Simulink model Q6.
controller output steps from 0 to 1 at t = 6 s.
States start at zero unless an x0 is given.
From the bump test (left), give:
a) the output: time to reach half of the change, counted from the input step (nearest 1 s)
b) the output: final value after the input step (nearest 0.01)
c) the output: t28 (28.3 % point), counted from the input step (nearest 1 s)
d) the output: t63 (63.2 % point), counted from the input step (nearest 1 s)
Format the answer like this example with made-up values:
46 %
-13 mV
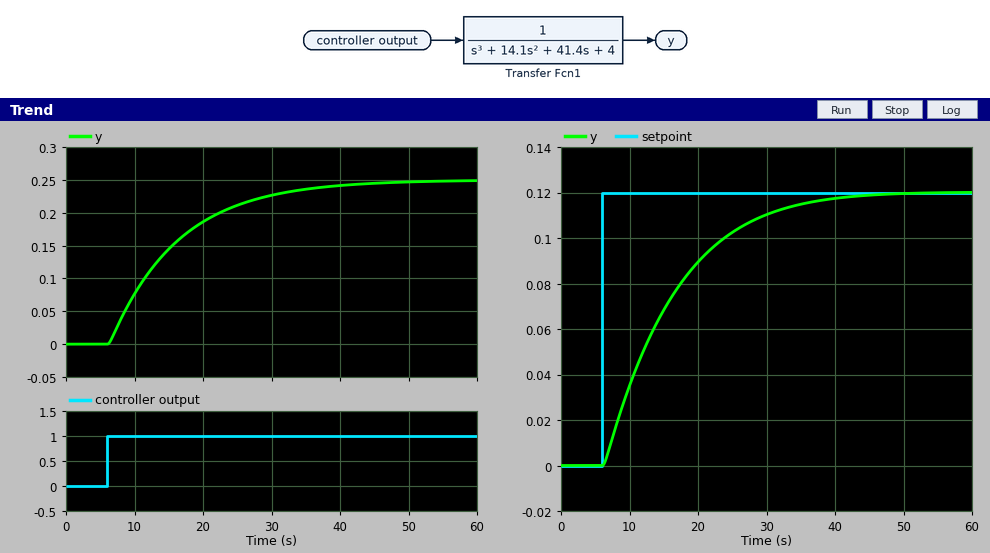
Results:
7 s
0.25
4 s
10 s
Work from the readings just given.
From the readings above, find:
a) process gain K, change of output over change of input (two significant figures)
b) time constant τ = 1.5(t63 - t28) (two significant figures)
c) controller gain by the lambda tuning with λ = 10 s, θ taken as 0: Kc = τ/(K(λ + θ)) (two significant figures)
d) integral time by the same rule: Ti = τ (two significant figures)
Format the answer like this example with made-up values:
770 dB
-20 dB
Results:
0.25
9.0 s
3.6
9.0 s
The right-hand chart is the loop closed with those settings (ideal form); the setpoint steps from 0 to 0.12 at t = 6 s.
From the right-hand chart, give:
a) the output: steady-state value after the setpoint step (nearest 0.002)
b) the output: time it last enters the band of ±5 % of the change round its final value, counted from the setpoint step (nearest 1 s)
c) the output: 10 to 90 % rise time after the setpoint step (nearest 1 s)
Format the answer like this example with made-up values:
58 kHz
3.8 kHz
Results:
0.120
28 s
21 s
